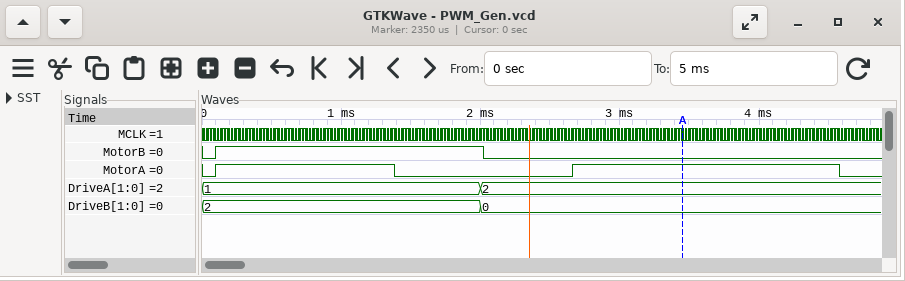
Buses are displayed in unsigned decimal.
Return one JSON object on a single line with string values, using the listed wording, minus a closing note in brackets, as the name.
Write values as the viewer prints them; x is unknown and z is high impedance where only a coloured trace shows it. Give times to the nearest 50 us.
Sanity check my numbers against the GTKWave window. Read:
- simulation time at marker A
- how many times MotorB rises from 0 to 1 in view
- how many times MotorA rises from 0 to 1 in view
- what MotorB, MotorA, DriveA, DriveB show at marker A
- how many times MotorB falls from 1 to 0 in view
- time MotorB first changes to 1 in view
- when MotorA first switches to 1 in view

{"simulation time at marker A": "3450 us", "how many times MotorB rises from 0 to 1 in view": "1", "how many times MotorA rises from 0 to 1 in view": "2", "what MotorB, MotorA, DriveA, DriveB show at marker A": "MotorB=0, MotorA=1, DriveA=2, DriveB=0", "how many times MotorB falls from 1 to 0 in view": "1", "time MotorB first changes to 1 in view": "100 us", "when MotorA first switches to 1 in view": "100 us"}
